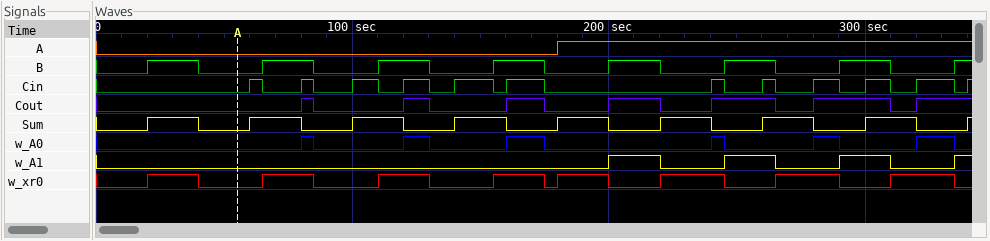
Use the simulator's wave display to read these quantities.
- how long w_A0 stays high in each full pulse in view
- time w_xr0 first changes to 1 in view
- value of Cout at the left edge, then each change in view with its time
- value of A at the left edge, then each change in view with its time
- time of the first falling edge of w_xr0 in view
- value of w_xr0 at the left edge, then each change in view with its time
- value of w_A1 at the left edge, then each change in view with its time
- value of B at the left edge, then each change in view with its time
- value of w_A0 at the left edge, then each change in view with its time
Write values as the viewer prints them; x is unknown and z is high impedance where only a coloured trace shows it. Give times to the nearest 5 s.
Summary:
5 s, 10 s, 15 s, 5 s, 10 s, 15 s
20 s
0, 1 at 80 s, 0 at 85 s, 1 at 120 s, 0 at 130 s, 1 at 160 s, 0 at 175 s, 1 at 200 s, 0 at 220 s, 1 at 240 s, 0 at 265 s, 1 at 280 s, 0 at 310 s, 1 at 320 s
0, 1 at 180 s
40 s
0, 1 at 20 s, 0 at 40 s, 1 at 65 s, 0 at 85 s, 1 at 110 s, 0 at 130 s, 1 at 155 s, 0 at 175 s, 1 at 180 s, 0 at 200 s, 1 at 220 s, 0 at 245 s, 1 at 265 s, 0 at 290 s, 1 at 310 s, 0 at 335 s
0, 1 at 200 s, 0 at 220 s, 1 at 245 s, 0 at 265 s, 1 at 290 s, 0 at 310 s, 1 at 335 s
0, 1 at 20 s, 0 at 40 s, 1 at 65 s, 0 at 85 s, 1 at 110 s, 0 at 130 s, 1 at 155 s, 0 at 175 s, 1 at 200 s, 0 at 220 s, 1 at 245 s, 0 at 265 s, 1 at 290 s, 0 at 310 s, 1 at 335 s
0, 1 at 80 s, 0 at 85 s, 1 at 120 s, 0 at 130 s, 1 at 160 s, 0 at 175 s, 1 at 240 s, 0 at 245 s, 1 at 280 s, 0 at 290 s, 1 at 320 s, 0 at 335 s
